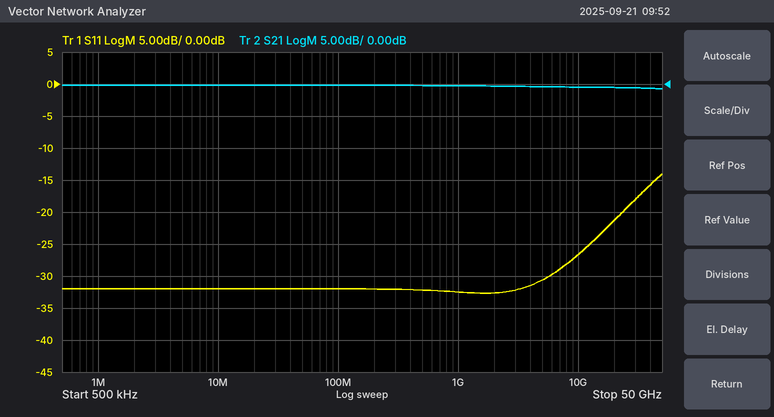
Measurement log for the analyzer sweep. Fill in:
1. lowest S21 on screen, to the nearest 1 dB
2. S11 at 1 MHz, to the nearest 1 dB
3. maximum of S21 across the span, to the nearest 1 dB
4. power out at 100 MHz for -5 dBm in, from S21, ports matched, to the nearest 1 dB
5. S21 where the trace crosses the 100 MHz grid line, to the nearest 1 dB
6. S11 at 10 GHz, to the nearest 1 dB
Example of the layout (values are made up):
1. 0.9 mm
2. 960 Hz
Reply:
1. -1 dB
2. -32 dB
3. 0 dB
4. -5 dBm
5. 0 dB
6. -27 dB
